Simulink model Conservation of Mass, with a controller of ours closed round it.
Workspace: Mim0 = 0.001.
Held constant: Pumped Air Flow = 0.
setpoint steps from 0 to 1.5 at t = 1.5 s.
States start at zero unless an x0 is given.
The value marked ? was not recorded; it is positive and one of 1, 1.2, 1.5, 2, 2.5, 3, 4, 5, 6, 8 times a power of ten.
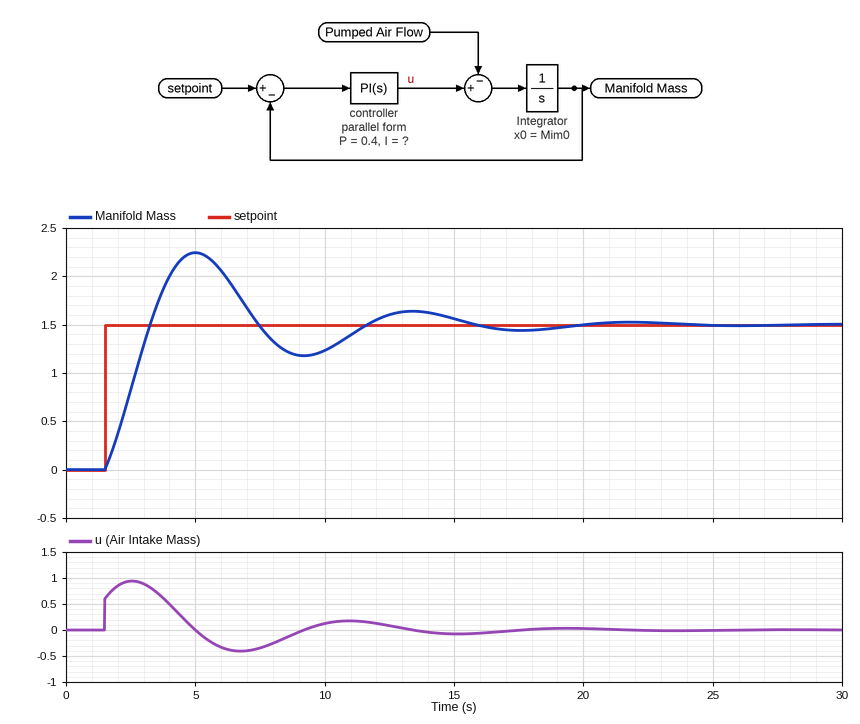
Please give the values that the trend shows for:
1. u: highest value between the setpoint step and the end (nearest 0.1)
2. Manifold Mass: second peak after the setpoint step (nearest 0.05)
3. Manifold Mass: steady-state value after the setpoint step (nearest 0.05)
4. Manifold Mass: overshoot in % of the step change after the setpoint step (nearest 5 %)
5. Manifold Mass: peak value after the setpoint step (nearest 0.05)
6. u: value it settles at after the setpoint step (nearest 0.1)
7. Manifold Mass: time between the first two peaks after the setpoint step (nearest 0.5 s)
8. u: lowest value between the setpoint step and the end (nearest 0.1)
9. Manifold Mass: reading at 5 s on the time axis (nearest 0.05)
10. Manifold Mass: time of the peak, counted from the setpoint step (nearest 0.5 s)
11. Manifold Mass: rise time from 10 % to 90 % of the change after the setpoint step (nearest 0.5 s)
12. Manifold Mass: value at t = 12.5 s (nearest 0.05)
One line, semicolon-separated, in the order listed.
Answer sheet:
0.9; 1.65; 1.50; 50 %; 2.25; 0.0; 8.5 s; -0.4; 2.25; 3.5 s; 1.5 s; 1.60
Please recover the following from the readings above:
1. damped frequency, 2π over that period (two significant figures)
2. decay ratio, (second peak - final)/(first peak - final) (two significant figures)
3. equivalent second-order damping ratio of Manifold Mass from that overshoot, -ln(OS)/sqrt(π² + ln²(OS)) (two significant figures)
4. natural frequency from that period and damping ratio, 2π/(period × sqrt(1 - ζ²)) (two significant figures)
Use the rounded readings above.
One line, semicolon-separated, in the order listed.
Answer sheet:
0.74 rad/s; 0.20; 0.22; 0.76 rad/s
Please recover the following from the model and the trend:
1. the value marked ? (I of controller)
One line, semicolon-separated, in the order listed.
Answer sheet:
0.6
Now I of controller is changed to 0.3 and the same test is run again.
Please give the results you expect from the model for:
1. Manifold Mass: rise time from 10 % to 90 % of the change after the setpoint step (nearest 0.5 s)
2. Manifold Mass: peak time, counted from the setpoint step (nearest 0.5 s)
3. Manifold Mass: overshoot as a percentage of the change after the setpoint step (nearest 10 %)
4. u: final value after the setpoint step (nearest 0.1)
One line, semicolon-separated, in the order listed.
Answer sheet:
2.0 s; 4.5 s; 40 %; 0.0
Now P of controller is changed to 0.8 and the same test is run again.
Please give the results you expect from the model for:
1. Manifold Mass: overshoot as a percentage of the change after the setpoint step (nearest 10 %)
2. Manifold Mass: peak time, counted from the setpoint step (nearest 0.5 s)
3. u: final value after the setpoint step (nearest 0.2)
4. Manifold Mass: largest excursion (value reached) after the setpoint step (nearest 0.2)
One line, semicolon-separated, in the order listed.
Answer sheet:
30 %; 3.0 s; 0.0; 2.0
